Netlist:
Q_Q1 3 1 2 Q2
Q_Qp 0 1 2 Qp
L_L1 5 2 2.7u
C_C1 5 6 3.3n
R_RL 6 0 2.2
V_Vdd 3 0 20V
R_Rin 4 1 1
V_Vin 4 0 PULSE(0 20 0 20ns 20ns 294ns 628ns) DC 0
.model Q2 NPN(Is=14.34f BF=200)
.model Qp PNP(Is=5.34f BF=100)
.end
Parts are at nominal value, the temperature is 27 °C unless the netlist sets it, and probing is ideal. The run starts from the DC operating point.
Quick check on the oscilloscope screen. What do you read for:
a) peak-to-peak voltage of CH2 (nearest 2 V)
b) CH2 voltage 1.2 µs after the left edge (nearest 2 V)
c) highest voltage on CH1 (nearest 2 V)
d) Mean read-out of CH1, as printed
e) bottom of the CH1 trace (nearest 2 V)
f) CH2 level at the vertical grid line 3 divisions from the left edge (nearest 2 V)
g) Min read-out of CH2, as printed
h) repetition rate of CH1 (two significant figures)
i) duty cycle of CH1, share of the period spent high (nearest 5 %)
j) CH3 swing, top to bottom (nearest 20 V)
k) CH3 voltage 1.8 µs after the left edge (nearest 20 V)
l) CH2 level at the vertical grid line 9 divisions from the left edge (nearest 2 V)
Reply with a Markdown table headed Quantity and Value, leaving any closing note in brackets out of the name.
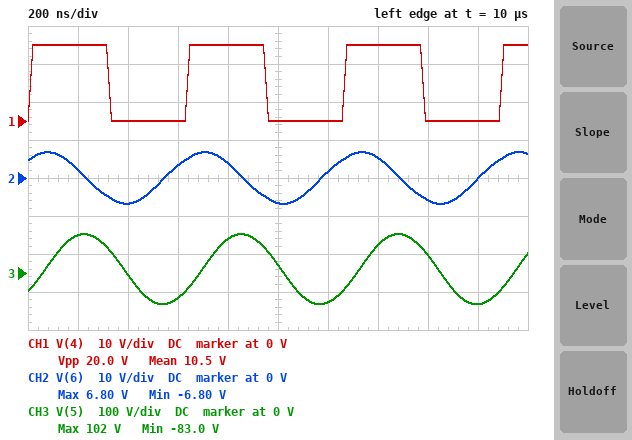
| Quantity | Value |
|---|---|
| peak-to-peak voltage of CH2 | 14 V |
| CH2 voltage 1.2 µs after the left edge | 2 V |
| highest voltage on CH1 | 20 V |
| Mean read-out of CH1, as printed | 10.5 V |
| bottom of the CH1 trace | 0 V |
| CH2 level at the vertical grid line 3 divisions from the left edge | 4 V |
| Min read-out of CH2, as printed | -6.80 V |
| repetition rate of CH1 | 1.6 MHz |
| duty cycle of CH1, share of the period spent high | 50 % |
| CH3 swing, top to bottom | 180 V |
| CH3 voltage 1.8 µs after the left edge | -80 V |
| CH2 level at the vertical grid line 9 divisions from the left edge | 0 V |
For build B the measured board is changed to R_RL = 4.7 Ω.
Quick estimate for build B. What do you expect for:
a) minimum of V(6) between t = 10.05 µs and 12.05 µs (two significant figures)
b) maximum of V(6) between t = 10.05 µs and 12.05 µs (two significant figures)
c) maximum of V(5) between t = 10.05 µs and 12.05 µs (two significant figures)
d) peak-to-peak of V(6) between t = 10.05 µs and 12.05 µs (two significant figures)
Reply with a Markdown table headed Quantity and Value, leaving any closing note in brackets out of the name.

| Quantity | Value |
|---|---|
| minimum of V(6) between t = 10.05 µs and 12.05 µs | -9.9 V |
| maximum of V(6) between t = 10.05 µs and 12.05 µs | 9.9 V |
| maximum of V(5) between t = 10.05 µs and 12.05 µs | 73 V |
| peak-to-peak of V(6) between t = 10.05 µs and 12.05 µs | 20 V |
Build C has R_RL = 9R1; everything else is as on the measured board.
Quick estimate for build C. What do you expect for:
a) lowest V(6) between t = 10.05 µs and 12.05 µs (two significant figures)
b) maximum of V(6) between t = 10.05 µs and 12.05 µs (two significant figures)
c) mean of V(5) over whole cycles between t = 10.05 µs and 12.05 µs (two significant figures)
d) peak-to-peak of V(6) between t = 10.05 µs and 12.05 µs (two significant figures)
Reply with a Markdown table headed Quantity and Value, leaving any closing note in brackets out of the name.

| Quantity | Value |
|---|---|
| lowest V(6) between t = 10.05 µs and 12.05 µs | -11 V |
| maximum of V(6) between t = 10.05 µs and 12.05 µs | 11 V |
| mean of V(5) over whole cycles between t = 10.05 µs and 12.05 µs | 10 V |
| peak-to-peak of V(6) between t = 10.05 µs and 12.05 µs | 23 V |
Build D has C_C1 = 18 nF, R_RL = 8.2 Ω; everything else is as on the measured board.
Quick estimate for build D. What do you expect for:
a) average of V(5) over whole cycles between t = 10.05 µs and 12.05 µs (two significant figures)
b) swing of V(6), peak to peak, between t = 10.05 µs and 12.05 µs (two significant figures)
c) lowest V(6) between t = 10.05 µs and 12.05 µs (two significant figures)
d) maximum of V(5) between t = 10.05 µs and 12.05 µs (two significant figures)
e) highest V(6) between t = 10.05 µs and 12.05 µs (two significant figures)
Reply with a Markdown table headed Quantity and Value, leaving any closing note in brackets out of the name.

| Quantity | Value |
|---|---|
| average of V(5) over whole cycles between t = 10.05 µs and 12.05 µs | 10 V |
| swing of V(6), peak to peak, between t = 10.05 µs and 12.05 µs | 9.6 V |
| lowest V(6) between t = 10.05 µs and 12.05 µs | -4.8 V |
| maximum of V(5) between t = 10.05 µs and 12.05 µs | 16 V |
| highest V(6) between t = 10.05 µs and 12.05 µs | 4.8 V |
